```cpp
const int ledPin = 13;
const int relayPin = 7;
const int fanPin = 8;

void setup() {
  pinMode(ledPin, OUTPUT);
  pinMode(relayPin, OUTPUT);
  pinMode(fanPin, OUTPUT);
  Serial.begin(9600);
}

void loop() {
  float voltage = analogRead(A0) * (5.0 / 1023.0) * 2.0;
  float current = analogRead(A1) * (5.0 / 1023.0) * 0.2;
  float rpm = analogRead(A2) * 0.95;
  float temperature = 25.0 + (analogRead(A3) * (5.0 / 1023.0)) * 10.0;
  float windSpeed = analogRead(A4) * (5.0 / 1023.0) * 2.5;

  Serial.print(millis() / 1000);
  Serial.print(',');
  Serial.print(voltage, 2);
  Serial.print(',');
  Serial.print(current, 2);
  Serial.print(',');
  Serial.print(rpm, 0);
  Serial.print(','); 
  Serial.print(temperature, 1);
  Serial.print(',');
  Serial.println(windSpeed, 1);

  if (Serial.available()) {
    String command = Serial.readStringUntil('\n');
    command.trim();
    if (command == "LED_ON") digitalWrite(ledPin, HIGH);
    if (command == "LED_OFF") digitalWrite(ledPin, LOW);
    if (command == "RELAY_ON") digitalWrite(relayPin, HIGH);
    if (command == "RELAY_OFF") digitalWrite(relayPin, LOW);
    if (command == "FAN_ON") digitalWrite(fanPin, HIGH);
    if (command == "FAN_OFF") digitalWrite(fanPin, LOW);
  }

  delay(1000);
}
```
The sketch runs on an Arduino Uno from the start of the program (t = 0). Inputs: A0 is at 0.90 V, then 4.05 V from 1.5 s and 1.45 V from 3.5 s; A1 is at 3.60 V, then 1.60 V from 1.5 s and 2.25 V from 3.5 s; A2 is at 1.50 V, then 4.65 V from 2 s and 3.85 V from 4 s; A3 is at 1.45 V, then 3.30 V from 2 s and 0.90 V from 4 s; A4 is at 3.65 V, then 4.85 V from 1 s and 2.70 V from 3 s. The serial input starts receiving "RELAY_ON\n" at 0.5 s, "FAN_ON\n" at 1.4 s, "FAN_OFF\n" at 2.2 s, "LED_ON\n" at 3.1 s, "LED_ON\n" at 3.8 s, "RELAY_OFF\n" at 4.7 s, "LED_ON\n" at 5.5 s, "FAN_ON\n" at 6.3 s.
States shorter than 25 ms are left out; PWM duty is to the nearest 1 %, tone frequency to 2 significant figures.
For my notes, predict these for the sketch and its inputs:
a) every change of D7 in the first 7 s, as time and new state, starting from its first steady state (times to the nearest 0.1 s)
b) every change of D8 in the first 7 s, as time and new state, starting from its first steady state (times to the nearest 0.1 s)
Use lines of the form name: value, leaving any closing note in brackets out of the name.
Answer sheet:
every change of D7 in the first 7 s, as time and new state, starting from its first steady state: 0 s low; 1 s high; 6 s low
every change of D8 in the first 7 s, as time and new state, starting from its first steady state: 0 s low; 2 s high; 3 s low
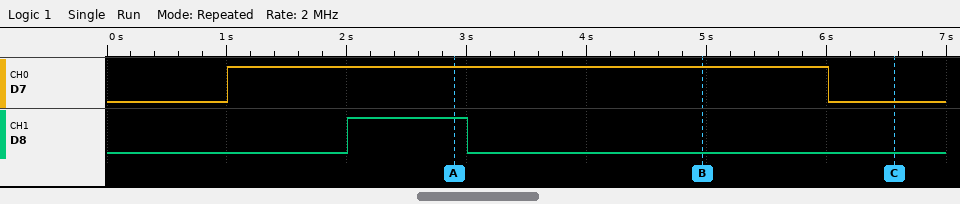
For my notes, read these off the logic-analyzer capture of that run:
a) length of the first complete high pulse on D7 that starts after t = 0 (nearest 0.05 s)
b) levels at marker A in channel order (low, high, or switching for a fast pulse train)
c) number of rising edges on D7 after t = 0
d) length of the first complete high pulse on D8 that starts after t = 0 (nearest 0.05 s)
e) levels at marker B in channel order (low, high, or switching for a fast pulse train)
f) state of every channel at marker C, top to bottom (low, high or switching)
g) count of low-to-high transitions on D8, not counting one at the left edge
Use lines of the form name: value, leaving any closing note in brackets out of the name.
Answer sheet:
length of the first complete high pulse on D7 that starts after t = 0: 5.00 s
levels at marker A in channel order: D7 high, D8 high
number of rising edges on D7 after t = 0: 1
length of the first complete high pulse on D8 that starts after t = 0: 1.00 s
levels at marker B in channel order: D7 high, D8 low
state of every channel at marker C, top to bottom: D7 low, D8 low
count of low-to-high transitions on D8, not counting one at the left edge: 1
